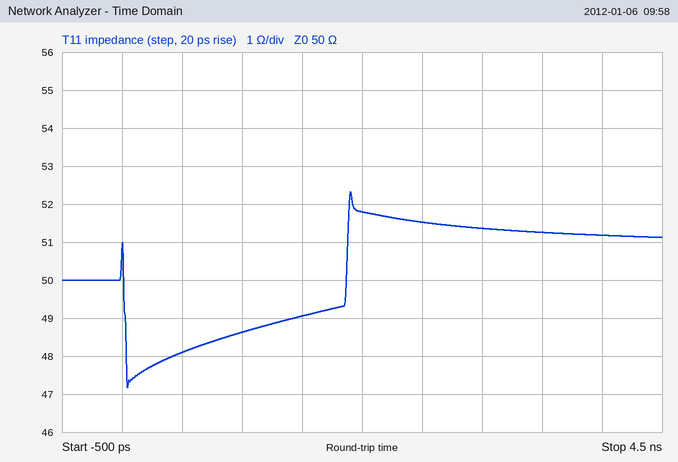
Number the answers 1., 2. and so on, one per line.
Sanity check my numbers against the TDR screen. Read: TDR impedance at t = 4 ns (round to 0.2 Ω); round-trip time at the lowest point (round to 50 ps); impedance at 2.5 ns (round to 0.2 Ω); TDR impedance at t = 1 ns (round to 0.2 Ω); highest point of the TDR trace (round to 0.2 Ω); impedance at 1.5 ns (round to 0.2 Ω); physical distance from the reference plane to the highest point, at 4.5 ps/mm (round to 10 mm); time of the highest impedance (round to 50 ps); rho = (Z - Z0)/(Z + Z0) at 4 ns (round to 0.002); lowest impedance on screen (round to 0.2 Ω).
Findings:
1. 51.2 Ω
2. 50 ps
3. 51.6 Ω
4. 48.6 Ω
5. 52.4 Ω
6. 49.0 Ω
7. 210 mm
8. 1.90 ns
9. +0.012
10. 47.2 Ω
